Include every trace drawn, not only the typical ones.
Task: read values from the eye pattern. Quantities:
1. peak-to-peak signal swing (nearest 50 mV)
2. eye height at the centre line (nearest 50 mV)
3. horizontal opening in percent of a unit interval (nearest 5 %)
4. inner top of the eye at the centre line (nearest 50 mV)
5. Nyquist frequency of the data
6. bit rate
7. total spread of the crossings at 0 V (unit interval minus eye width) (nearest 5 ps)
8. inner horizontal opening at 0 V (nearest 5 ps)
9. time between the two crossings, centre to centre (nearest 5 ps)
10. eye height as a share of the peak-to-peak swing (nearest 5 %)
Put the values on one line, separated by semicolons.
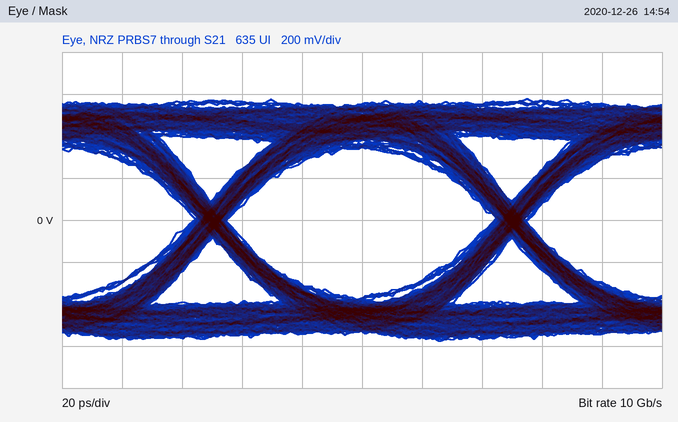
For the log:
1.15 V; 700 mV; 90 %; 350 mV; 5 GHz; 10 Gb/s; 10 ps; 90 ps; 100 ps; 60 %
